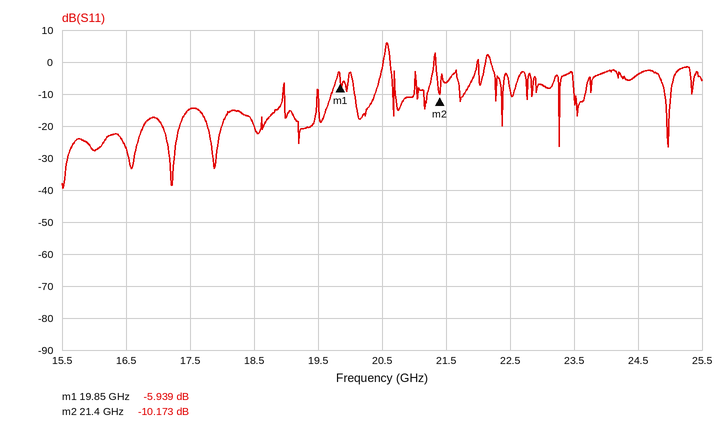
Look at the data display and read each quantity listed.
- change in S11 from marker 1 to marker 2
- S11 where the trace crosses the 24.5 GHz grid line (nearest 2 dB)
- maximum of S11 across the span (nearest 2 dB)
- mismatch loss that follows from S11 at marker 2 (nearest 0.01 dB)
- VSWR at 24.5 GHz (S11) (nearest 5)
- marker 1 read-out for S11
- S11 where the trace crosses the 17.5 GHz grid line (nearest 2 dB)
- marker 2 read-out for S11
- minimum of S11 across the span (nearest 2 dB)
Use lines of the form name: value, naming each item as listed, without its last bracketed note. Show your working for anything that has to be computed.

change in S11 from marker 1 to marker 2: -10.173 − (-5.939) = -4.234 dB
S11 where the trace crosses the 24.5 GHz grid line: -4 dB
maximum of S11 across the span: 6 dB
mismatch loss that follows from S11 at marker 2: −10 log10(1 − 10^(-10.173/10)) ≈ 0.44 dB
VSWR at 24.5 GHz (S11): |Γ| = 10^(-4/20) = 0.6310; VSWR = (1 + 0.6310)/(1 − 0.6310) ≈ 4.42, so 5 to the nearest 5
marker 1 read-out for S11: -5.939 dB
S11 where the trace crosses the 17.5 GHz grid line: -14 dB
marker 2 read-out for S11: -10.173 dB
minimum of S11 across the span: -40 dB
